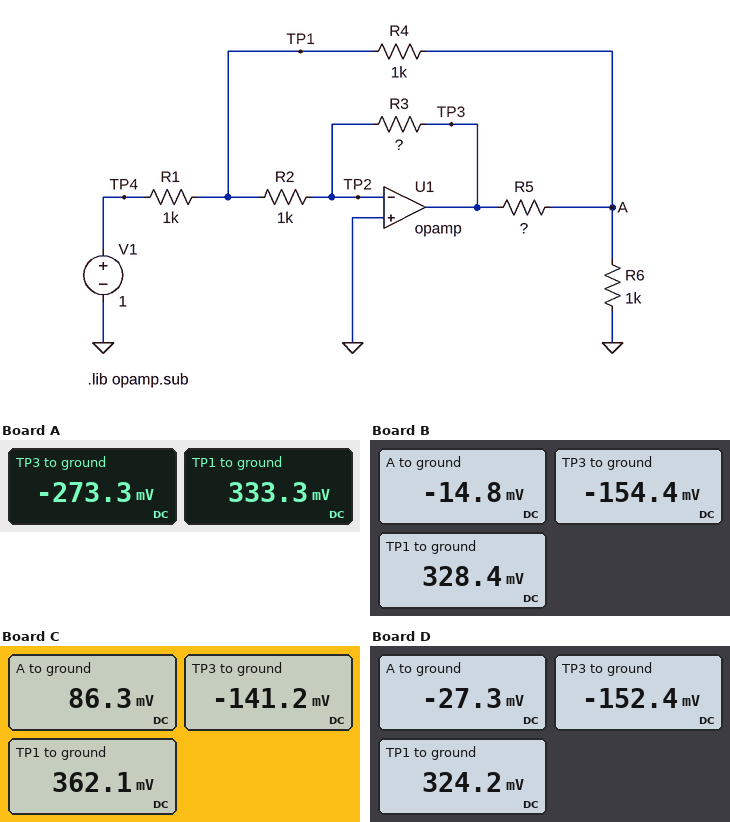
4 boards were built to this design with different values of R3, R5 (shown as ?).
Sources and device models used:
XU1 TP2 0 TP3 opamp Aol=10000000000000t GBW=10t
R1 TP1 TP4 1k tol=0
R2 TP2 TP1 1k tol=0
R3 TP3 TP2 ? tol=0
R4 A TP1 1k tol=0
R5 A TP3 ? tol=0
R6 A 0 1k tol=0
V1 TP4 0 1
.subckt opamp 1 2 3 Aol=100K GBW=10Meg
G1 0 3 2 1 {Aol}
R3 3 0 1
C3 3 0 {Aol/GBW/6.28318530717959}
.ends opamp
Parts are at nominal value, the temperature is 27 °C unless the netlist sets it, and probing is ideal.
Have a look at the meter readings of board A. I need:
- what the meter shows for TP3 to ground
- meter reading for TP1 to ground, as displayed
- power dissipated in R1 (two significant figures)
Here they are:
-273.3 mV
333.3 mV
440 µW
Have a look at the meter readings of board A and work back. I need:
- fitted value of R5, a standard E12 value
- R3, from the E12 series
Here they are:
820 Ω
820 Ω
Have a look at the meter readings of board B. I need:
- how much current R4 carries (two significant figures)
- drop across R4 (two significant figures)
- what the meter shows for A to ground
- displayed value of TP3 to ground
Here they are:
340 µA
340 mV
-14.8 mV
-154.4 mV
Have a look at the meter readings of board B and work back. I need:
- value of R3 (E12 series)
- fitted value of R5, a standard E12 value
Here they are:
470 Ω
390 Ω
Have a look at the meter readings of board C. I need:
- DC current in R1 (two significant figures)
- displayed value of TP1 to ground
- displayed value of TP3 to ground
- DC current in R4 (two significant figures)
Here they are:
640 µA
362.1 mV
-141.2 mV
280 µA
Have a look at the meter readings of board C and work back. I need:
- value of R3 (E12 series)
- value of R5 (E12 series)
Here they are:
390 Ω
1.2 kΩ
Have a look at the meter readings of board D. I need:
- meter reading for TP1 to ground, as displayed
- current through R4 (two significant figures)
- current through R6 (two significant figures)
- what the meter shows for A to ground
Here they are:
324.2 mV
350 µA
27 µA
-27.3 mV
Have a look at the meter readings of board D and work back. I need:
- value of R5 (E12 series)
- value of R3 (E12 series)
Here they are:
330 Ω
470 Ω
